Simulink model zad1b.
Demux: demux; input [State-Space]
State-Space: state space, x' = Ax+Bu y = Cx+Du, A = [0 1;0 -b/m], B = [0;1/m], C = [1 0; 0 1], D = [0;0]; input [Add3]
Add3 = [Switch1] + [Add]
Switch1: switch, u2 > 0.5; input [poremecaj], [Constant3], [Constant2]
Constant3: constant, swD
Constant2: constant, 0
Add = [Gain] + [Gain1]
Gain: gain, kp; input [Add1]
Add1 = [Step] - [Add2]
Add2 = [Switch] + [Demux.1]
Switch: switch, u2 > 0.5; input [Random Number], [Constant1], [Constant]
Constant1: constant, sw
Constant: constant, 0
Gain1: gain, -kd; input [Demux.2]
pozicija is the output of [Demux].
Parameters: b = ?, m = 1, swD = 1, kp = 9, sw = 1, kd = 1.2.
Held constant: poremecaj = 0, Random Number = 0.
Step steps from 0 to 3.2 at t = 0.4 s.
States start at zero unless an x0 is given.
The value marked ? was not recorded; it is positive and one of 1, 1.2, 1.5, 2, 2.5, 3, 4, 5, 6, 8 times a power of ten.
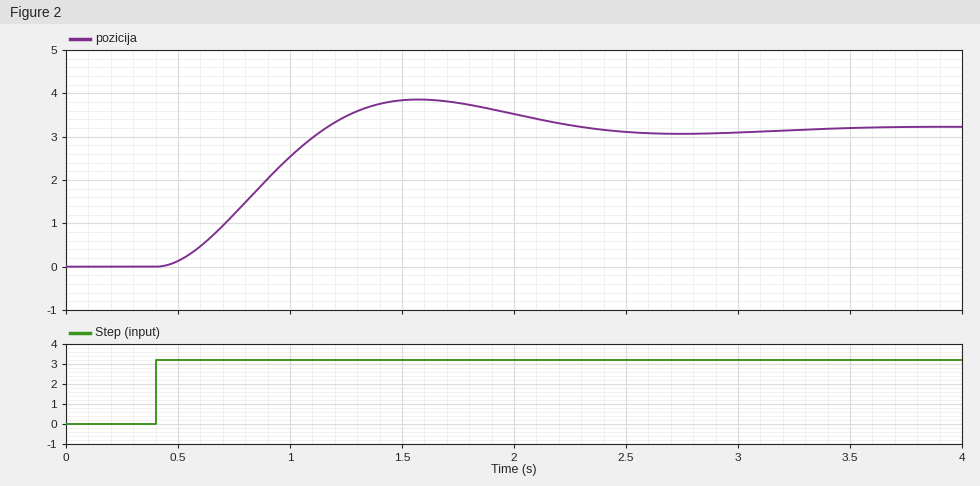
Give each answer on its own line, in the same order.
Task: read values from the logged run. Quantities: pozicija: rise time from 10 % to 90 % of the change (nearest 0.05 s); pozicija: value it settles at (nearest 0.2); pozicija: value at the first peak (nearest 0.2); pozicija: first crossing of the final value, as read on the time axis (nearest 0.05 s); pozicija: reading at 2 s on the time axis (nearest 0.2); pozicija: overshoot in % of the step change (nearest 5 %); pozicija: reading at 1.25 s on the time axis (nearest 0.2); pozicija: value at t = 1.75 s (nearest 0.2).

0.50 s
3.2
3.8
1.15 s
3.6
20 %
3.4
3.8
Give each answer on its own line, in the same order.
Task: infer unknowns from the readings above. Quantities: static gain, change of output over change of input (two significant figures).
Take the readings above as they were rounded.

1.0
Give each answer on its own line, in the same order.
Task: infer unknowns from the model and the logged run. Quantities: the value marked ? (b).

1.5
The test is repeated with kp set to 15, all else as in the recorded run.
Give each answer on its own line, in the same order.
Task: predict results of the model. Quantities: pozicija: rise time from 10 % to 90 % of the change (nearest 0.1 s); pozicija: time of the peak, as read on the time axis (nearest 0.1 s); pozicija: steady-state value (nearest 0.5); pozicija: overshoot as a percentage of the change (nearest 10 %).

0.4 s
1.3 s
3.0
30 %
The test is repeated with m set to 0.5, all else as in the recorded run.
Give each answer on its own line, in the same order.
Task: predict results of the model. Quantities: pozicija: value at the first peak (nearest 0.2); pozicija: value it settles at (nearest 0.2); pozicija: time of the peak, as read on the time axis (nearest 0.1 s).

3.4
3.2
1.4 s
